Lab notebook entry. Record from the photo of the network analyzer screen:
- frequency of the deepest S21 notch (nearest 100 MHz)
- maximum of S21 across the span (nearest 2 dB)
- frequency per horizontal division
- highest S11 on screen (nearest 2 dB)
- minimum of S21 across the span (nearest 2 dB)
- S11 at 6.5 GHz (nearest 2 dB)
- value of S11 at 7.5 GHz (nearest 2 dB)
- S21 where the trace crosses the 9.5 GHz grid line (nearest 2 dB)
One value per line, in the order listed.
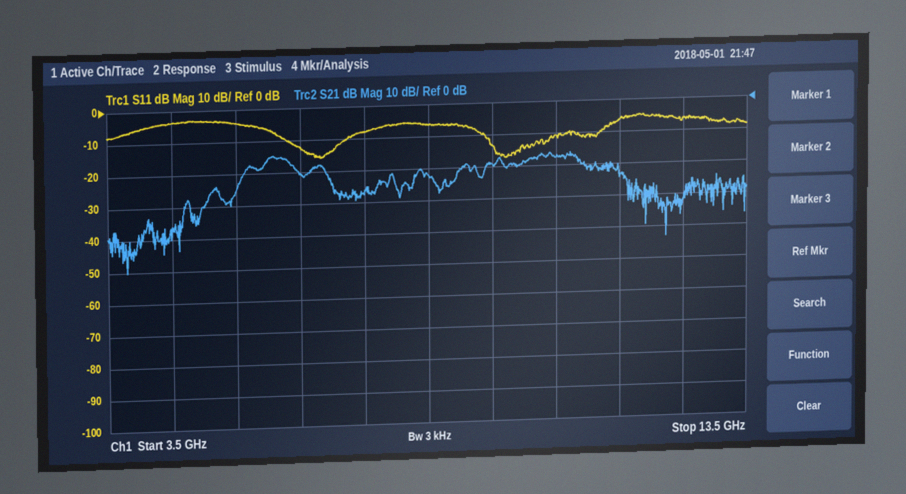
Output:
3.8 GHz
-14 dB
1 GHz
-4 dB
-50 dB
-12 dB
-8 dB
-20 dB
